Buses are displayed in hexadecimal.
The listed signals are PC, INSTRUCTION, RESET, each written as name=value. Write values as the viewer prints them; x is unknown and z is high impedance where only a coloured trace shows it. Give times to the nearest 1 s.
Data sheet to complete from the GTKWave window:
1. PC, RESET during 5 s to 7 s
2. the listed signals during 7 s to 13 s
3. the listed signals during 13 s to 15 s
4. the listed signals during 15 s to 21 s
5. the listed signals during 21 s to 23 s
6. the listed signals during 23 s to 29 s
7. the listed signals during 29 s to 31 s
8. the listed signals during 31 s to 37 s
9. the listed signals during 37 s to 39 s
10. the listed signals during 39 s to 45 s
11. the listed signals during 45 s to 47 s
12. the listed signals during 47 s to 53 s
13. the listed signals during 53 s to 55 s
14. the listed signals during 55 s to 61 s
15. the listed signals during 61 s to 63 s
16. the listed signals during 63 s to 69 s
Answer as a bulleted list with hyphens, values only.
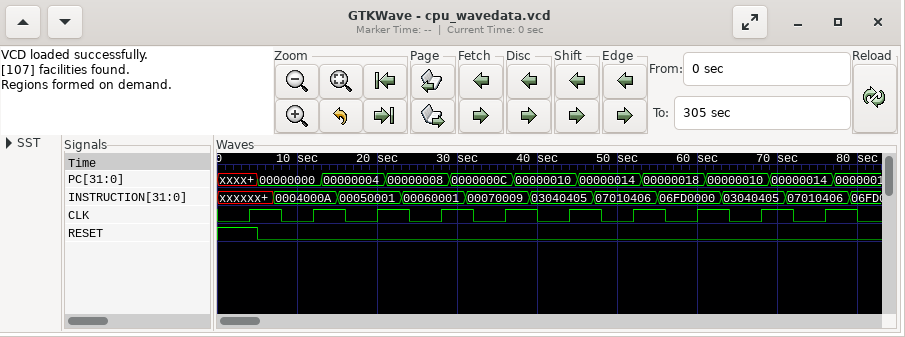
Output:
- PC=00000000, RESET=0
- PC=00000000, INSTRUCTION=0004000A, RESET=0
- PC=00000004, INSTRUCTION=0004000A, RESET=0
- PC=00000004, INSTRUCTION=00050001, RESET=0
- PC=00000008, INSTRUCTION=00050001, RESET=0
- PC=00000008, INSTRUCTION=00060001, RESET=0
- PC=0000000C, INSTRUCTION=00060001, RESET=0
- PC=0000000C, INSTRUCTION=00070009, RESET=0
- PC=00000010, INSTRUCTION=00070009, RESET=0
- PC=00000010, INSTRUCTION=03040405, RESET=0
- PC=00000014, INSTRUCTION=03040405, RESET=0
- PC=00000014, INSTRUCTION=07010406, RESET=0
- PC=00000018, INSTRUCTION=07010406, RESET=0
- PC=00000018, INSTRUCTION=06FD0000, RESET=0
- PC=00000010, INSTRUCTION=06FD0000, RESET=0
- PC=00000010, INSTRUCTION=03040405, RESET=0
